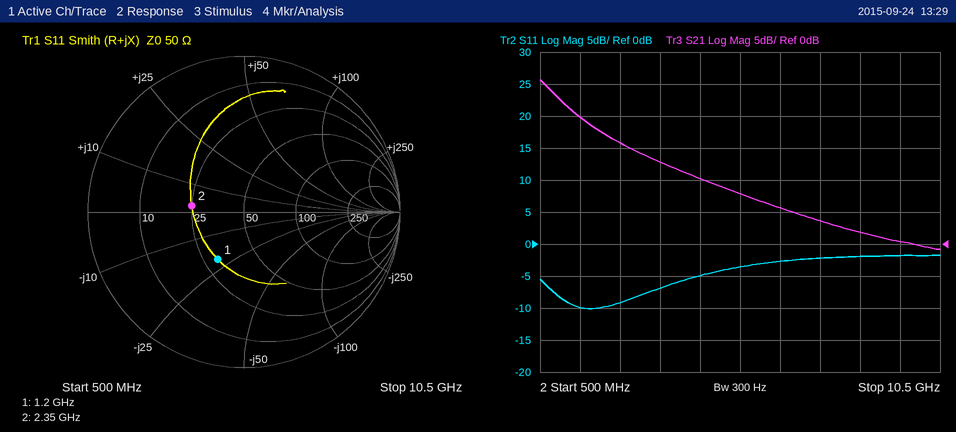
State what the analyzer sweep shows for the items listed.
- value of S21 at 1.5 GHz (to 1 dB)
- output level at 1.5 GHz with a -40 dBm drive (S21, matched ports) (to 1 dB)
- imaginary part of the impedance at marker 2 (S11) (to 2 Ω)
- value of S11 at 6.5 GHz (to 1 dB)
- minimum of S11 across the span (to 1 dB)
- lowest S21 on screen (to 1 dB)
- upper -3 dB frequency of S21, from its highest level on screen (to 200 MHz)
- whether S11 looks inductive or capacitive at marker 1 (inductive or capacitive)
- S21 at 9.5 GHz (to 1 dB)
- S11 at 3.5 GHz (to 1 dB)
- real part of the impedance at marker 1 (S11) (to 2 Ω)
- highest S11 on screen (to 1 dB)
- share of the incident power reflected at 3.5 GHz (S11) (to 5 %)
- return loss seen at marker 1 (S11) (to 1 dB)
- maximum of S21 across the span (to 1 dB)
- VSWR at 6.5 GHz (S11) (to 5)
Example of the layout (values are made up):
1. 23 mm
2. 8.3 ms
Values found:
1. 20 dB
2. -20 dBm
3. +2 Ω
4. -3 dB
5. -10 dB
6. -1 dB
7. 1.0 GHz
8. capacitive
9. 0 dB
10. -7 dB
11. 30 Ω
12. -2 dB
13. 20 %
14. 9 dB
15. 26 dB
16. 5
